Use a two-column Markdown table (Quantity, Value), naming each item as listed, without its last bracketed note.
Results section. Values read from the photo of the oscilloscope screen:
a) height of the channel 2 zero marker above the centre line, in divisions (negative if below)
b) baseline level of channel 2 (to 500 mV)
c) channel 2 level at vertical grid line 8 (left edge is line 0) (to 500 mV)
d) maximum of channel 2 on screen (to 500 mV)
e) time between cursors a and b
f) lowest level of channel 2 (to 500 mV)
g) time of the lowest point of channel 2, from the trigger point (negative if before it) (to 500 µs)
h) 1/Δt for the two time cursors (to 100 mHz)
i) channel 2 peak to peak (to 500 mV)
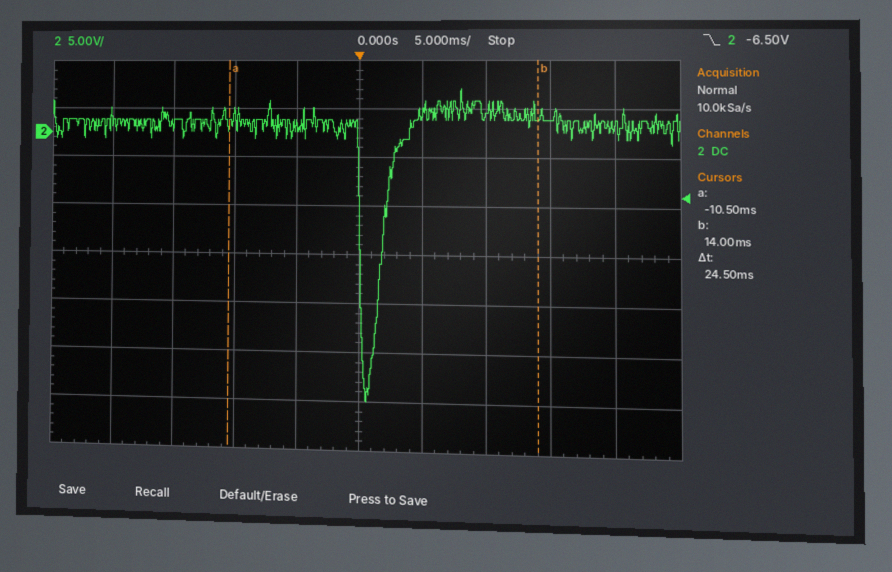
| Quantity | Value |
|---|---|
| height of the channel 2 zero marker above the centre line, in divisions | +2.5 div |
| baseline level of channel 2 | 1.0 V |
| channel 2 level at vertical grid line 8 (left edge is line 0) | 1.5 V |
| maximum of channel 2 on screen | 4.5 V |
| time between cursors a and b | 24.5 ms |
| lowest level of channel 2 | -27.5 V |
| time of the lowest point of channel 2, from the trigger point (negative if before it) | +500 µs |
| 1/Δt for the two time cursors | 40.8 Hz |
| channel 2 peak to peak | 32.0 V |
